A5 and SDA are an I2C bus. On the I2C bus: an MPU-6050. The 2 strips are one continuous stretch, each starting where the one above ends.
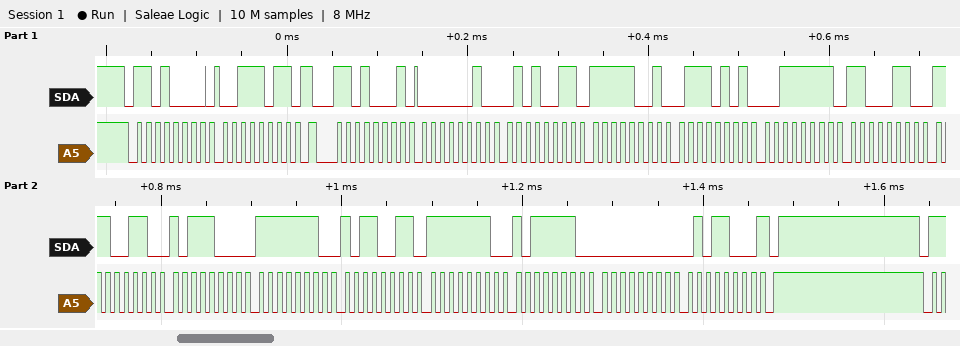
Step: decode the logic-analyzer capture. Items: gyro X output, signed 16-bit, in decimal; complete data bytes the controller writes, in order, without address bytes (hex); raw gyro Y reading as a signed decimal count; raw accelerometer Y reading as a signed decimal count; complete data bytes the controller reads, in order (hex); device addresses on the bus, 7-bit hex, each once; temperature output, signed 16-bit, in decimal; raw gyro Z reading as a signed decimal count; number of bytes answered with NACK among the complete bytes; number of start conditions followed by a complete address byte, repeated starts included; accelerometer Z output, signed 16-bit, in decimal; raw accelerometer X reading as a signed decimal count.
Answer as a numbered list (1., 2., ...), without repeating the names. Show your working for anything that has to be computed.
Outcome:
1. 0xFEB3 = -333
2. 3B
3. 0xFEBE = -322
4. 0xF975 = -1675
5. 02 53 F9 75 3F C6 E6 B8 FE B3 FE BE 00 58
6. 0x68
7. 0xE6B8 = -6472
8. 0x0058 = 88
9. 1
10. 2
11. 0x3FC6 = 16326
12. 0x0253 = 595
